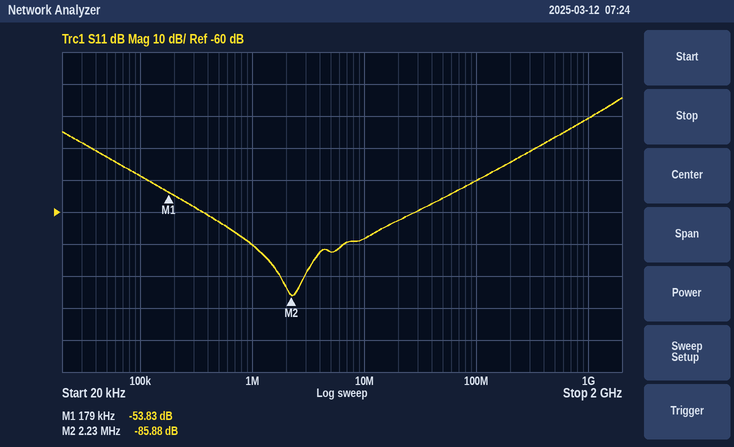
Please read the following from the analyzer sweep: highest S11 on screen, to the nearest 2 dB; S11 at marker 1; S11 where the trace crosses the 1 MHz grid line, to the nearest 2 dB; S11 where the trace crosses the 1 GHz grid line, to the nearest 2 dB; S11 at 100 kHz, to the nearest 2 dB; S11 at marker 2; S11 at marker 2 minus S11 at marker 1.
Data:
-24 dB
-53.83 dB
-70 dB
-30 dB
-48 dB
-85.88 dB
-32.05 dB
